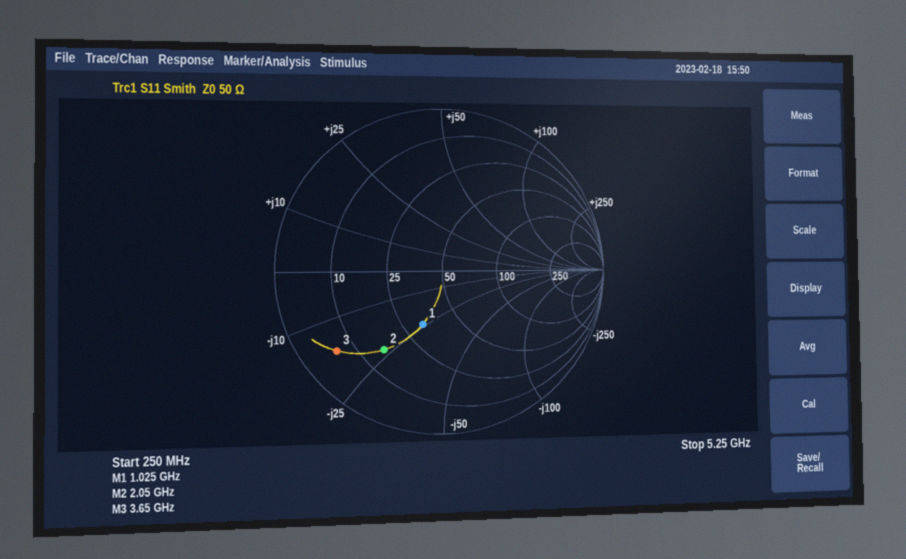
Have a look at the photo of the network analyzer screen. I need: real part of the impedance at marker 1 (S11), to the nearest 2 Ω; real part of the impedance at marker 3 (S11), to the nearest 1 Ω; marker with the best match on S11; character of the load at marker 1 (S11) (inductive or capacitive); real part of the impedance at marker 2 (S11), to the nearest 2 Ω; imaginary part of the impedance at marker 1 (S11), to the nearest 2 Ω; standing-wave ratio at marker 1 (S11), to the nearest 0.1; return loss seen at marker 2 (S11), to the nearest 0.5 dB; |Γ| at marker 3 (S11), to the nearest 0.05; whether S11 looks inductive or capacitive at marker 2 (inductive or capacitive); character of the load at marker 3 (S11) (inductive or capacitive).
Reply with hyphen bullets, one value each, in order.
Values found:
- 32 Ω
- 6 Ω
- marker 1
- capacitive
- 16 Ω
- -24 Ω
- 2.1
- 4.5 dB
- 0.80
- capacitive
- capacitive
